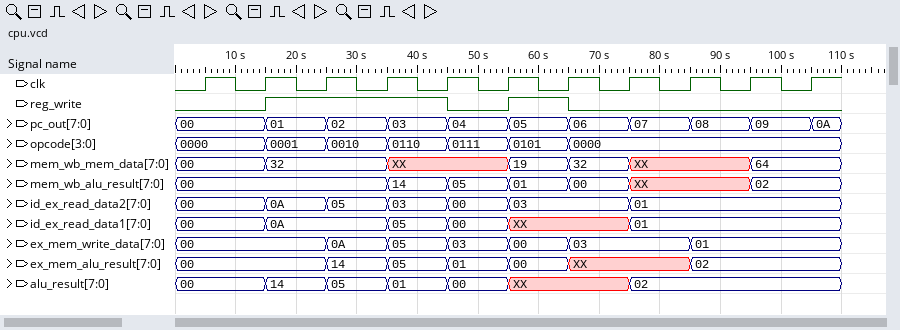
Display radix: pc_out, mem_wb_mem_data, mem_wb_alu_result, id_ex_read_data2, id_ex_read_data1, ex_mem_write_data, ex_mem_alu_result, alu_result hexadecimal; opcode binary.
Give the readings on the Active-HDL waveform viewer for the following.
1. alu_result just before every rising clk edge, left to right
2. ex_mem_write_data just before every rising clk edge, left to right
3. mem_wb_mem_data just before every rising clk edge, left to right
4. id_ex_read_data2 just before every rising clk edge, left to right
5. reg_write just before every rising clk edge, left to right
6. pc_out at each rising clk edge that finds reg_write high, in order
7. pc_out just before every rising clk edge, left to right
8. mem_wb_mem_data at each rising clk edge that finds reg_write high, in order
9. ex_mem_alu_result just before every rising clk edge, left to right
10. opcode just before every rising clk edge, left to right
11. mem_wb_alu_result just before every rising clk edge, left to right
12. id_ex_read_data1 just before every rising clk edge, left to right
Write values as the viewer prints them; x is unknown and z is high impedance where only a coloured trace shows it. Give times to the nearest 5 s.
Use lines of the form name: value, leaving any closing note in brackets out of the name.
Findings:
alu_result just before every rising clk edge, left to right: 00, 00, 14, 05, 01, 00, XX, XX, 02, 02, 02
ex_mem_write_data just before every rising clk edge, left to right: 00, 00, 00, 0A, 05, 03, 00, 03, 03, 01, 01
mem_wb_mem_data just before every rising clk edge, left to right: 00, 00, 32, 32, XX, XX, 19, 32, XX, XX, 64
id_ex_read_data2 just before every rising clk edge, left to right: 00, 00, 0A, 05, 03, 00, 03, 03, 01, 01, 01
reg_write just before every rising clk edge, left to right: 0 0 1 1 1 0 1 0 0 0 0
pc_out at each rising clk edge that finds reg_write high, in order: 01, 02, 03, 05
pc_out just before every rising clk edge, left to right: 00, 00, 01, 02, 03, 04, 05, 06, 07, 08, 09
mem_wb_mem_data at each rising clk edge that finds reg_write high, in order: 32, 32, XX, 19
ex_mem_alu_result just before every rising clk edge, left to right: 00, 00, 00, 14, 05, 01, 00, XX, XX, 02, 02
opcode just before every rising clk edge, left to right: 0000, 0000, 0001, 0010, 0110, 0111, 0101, 0000, 0000, 0000, 0000
mem_wb_alu_result just before every rising clk edge, left to right: 00, 00, 00, 00, 14, 05, 01, 00, XX, XX, 02
id_ex_read_data1 just before every rising clk edge, left to right: 00, 00, 0A, 0A, 05, 00, XX, XX, 01, 01, 01
